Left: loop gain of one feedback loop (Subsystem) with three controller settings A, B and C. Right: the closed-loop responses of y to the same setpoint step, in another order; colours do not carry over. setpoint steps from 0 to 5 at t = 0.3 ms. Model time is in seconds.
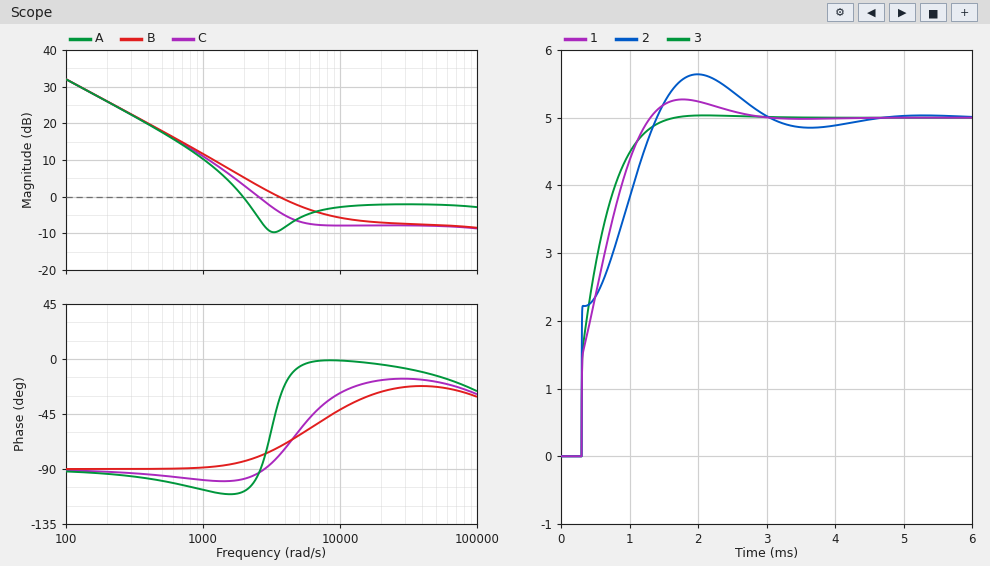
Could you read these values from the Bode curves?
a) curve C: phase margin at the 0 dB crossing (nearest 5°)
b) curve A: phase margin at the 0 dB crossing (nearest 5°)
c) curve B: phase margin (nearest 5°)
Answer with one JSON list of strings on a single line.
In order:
["85°", "70°", "110°"]
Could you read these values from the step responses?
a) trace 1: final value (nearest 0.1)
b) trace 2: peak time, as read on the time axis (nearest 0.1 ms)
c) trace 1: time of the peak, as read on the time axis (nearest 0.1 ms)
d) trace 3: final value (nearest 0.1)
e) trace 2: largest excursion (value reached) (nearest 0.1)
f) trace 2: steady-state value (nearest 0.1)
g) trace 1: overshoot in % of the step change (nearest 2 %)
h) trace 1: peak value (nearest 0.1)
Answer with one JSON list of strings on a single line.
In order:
["5.0", "2.0 ms", "1.8 ms", "5.0", "5.6", "5.0", "6 %", "5.3"]
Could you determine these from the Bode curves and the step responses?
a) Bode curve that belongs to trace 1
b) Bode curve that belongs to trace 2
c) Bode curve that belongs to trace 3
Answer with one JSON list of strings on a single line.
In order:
["C", "A", "B"]
